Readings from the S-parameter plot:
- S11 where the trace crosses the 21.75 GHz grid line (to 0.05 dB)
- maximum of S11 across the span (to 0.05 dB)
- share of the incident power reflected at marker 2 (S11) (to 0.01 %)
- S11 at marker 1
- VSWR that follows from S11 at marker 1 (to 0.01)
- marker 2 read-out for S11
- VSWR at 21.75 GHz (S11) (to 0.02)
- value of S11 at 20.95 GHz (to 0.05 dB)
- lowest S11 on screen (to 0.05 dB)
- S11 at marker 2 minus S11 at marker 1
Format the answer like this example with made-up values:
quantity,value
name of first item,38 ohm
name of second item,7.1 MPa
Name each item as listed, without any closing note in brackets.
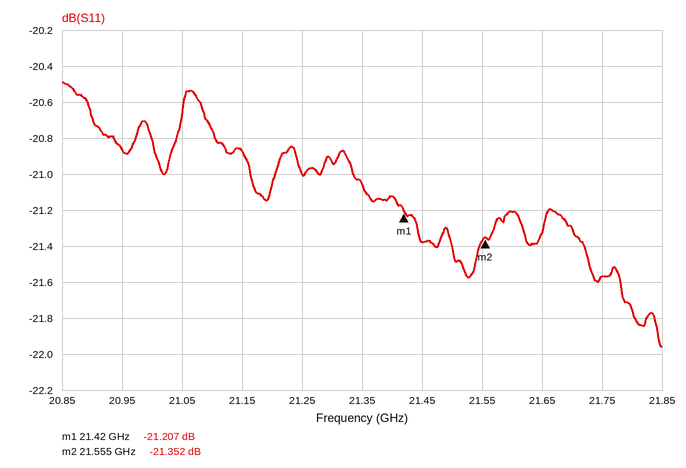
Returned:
quantity,value
S11 where the trace crosses the 21.75 GHz grid line,-21.55 dB
maximum of S11 across the span,-20.50 dB
share of the incident power reflected at marker 2 (S11),0.73 %
S11 at marker 1,-21.207 dB
VSWR that follows from S11 at marker 1,1.19
marker 2 read-out for S11,-21.352 dB
VSWR at 21.75 GHz (S11),1.18
value of S11 at 20.95 GHz,-20.85 dB
lowest S11 on screen,-21.95 dB
S11 at marker 2 minus S11 at marker 1,-0.145 dB
